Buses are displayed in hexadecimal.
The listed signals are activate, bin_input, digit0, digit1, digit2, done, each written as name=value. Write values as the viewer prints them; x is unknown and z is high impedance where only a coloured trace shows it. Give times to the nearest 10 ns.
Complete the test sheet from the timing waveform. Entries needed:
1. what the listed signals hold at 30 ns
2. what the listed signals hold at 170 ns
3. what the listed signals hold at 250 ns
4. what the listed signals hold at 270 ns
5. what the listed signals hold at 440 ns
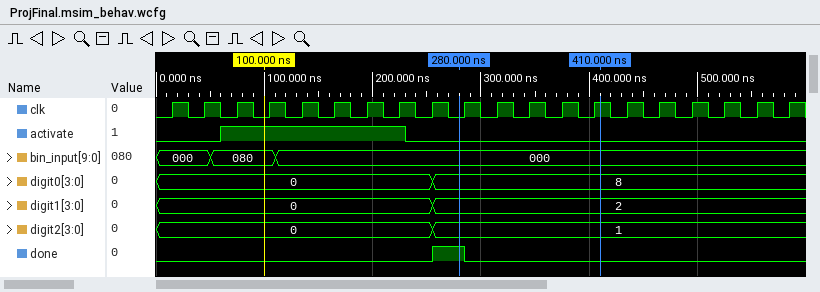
activate=0, bin_input=000, digit0=0, digit1=0, digit2=0, done=0
activate=1, bin_input=000, digit0=0, digit1=0, digit2=0, done=0
activate=0, bin_input=000, digit0=0, digit1=0, digit2=0, done=0
activate=0, bin_input=000, digit0=8, digit1=2, digit2=1, done=1
activate=0, bin_input=000, digit0=8, digit1=2, digit2=1, done=0
